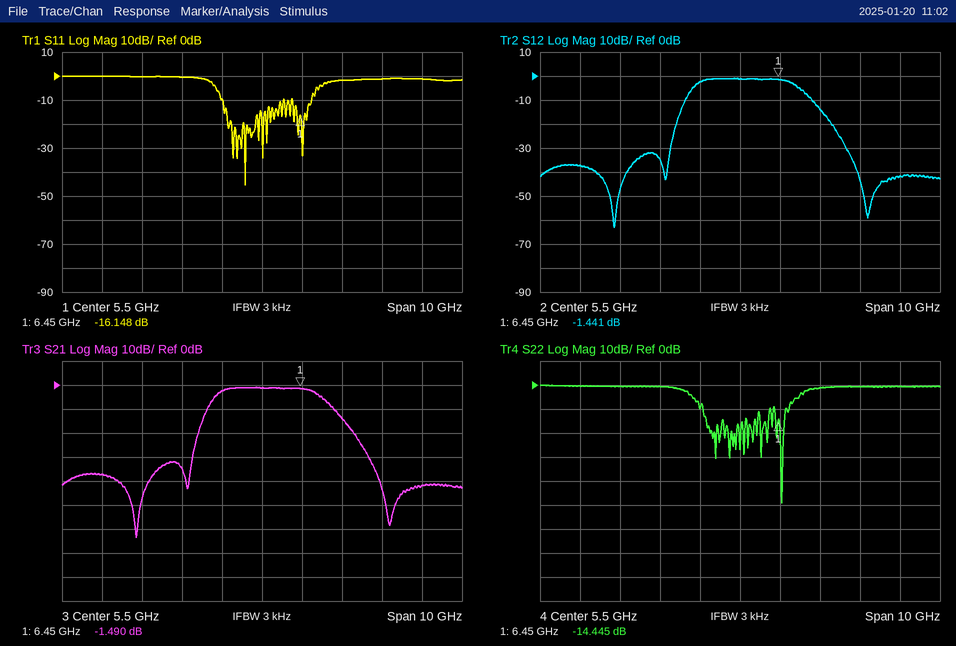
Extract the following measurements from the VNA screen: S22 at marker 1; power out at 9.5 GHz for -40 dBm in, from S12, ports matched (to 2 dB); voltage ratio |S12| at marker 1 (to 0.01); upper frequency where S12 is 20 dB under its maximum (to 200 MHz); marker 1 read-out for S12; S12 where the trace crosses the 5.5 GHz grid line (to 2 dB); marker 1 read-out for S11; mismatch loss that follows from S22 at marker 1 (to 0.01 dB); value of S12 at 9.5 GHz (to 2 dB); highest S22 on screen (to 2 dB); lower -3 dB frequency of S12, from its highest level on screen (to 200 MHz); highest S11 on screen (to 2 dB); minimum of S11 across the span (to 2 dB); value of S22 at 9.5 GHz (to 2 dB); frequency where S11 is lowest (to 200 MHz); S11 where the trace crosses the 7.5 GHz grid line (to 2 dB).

-14.445 dB
-82 dBm
0.85
7.8 GHz
-1.441 dB
-2 dB
-16.148 dB
0.16 dB
-42 dB
0 dB
4.4 GHz
0 dB
-46 dB
0 dB
5.0 GHz
-2 dB
